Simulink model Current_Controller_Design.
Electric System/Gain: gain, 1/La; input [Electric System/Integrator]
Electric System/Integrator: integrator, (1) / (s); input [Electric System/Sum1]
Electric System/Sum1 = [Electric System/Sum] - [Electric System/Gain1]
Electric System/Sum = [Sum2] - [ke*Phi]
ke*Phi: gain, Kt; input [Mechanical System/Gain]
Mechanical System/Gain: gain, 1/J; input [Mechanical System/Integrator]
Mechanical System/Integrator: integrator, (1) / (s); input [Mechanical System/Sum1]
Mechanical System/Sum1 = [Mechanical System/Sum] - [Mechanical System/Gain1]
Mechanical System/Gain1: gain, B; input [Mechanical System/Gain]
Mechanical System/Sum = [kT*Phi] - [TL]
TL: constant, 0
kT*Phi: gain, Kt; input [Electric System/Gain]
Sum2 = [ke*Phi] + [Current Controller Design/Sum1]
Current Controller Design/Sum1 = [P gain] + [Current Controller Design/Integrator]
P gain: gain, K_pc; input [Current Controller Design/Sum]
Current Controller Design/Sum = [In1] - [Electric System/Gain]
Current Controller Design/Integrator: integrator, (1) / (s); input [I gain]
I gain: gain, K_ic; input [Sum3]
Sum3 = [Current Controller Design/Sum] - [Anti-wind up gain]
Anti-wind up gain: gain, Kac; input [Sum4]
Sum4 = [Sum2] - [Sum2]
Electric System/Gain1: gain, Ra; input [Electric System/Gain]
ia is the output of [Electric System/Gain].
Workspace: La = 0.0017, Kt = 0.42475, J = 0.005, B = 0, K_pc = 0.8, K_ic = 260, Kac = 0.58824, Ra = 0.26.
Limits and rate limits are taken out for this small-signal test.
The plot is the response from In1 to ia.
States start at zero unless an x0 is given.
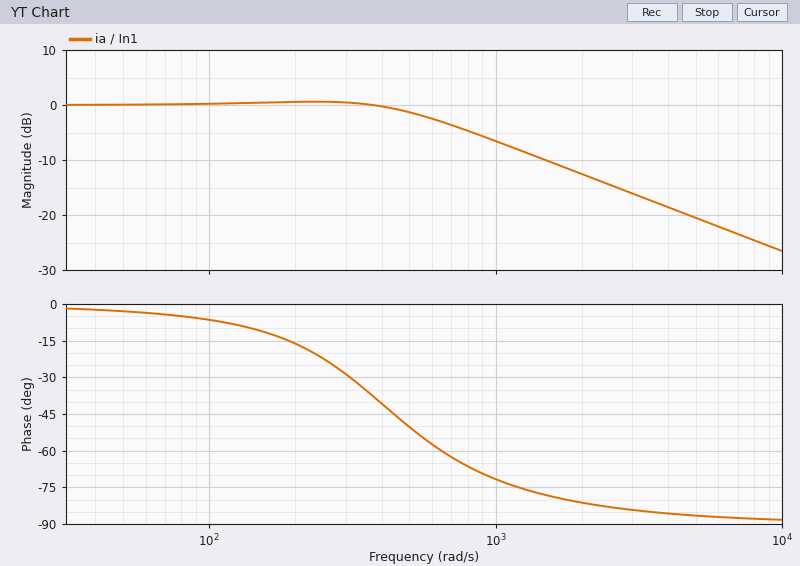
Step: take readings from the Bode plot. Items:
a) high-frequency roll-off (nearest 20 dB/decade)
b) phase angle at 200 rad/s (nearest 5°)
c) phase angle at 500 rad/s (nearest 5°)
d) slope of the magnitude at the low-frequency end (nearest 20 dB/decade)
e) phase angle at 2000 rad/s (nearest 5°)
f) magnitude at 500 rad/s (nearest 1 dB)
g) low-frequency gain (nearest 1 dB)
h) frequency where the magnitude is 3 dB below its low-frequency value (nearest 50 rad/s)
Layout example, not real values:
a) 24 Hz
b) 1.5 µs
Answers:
a) -20 dB/decade
b) -15°
c) -50°
d) 0 dB/decade
e) -80°
f) -1 dB
g) 0 dB
h) 650 rad/s
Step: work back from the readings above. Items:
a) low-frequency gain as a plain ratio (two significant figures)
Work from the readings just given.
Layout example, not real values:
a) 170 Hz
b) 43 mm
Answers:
a) 1.0
